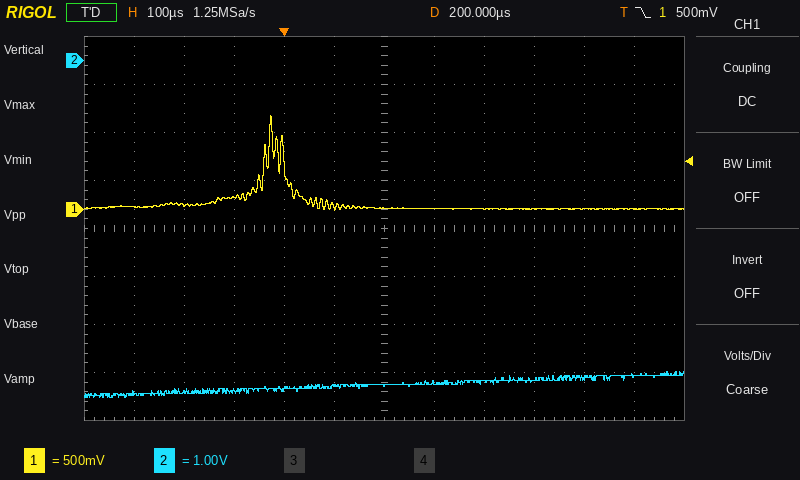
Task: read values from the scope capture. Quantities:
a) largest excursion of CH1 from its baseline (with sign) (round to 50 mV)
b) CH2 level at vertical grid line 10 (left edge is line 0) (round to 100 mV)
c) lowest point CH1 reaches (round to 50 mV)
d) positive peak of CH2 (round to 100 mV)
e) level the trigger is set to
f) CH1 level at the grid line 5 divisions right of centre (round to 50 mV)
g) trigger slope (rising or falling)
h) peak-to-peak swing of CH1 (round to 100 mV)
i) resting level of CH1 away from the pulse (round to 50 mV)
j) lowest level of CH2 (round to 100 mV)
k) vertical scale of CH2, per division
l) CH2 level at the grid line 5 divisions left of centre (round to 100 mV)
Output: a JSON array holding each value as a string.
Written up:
["+950 mV", "-6.6 V", "0 mV", "-6.5 V", "500 mV", "0 mV", "falling", "1.00 V", "0 mV", "-7.0 V", "1 V", "-6.9 V"]
